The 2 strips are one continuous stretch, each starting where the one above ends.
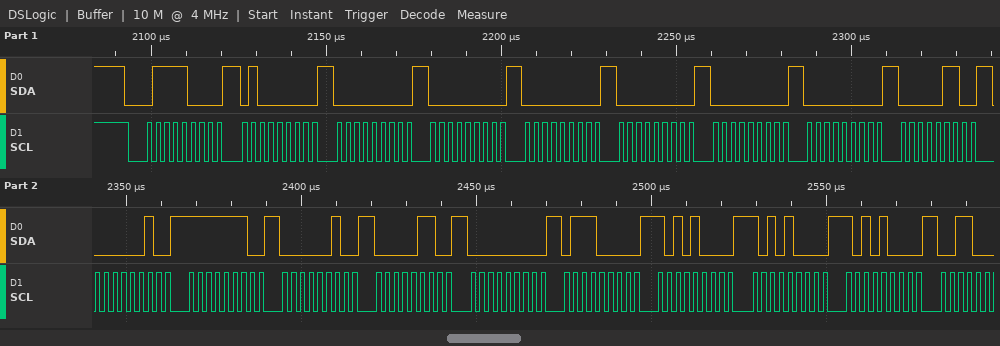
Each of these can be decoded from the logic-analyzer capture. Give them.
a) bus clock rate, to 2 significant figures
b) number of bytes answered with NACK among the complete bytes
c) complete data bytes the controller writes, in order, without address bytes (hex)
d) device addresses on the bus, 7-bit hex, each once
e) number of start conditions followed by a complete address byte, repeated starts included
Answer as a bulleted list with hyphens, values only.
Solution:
- 400 kHz
- 0
- 40 00 00 00 00 00 00 06 02 FE 02 06 00 70 A8 A8 A8
- 0x3C
- 1
